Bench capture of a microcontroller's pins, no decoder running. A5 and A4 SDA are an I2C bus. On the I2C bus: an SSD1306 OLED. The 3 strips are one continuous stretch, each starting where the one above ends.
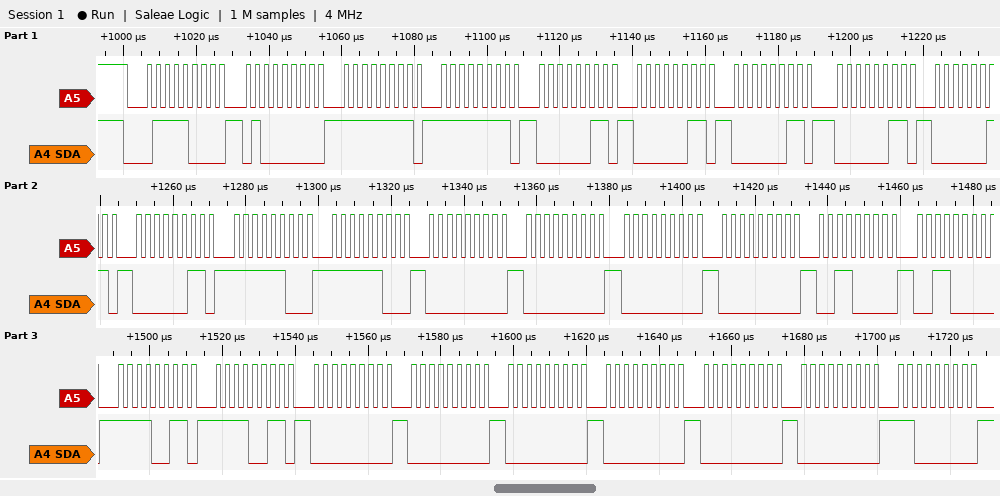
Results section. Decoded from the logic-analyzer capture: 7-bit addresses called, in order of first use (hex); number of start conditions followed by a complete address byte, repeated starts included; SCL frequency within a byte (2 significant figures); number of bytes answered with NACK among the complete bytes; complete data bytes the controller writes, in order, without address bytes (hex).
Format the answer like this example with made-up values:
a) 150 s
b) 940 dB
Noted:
a) 0x3C
b) 1
c) 400 kHz
d) 0
e) 40 FF FF 03 03 03 03 03 03 FC FC 00 00 00 00 30 30 F3 F3 00 00 00 00 00 00 C0
